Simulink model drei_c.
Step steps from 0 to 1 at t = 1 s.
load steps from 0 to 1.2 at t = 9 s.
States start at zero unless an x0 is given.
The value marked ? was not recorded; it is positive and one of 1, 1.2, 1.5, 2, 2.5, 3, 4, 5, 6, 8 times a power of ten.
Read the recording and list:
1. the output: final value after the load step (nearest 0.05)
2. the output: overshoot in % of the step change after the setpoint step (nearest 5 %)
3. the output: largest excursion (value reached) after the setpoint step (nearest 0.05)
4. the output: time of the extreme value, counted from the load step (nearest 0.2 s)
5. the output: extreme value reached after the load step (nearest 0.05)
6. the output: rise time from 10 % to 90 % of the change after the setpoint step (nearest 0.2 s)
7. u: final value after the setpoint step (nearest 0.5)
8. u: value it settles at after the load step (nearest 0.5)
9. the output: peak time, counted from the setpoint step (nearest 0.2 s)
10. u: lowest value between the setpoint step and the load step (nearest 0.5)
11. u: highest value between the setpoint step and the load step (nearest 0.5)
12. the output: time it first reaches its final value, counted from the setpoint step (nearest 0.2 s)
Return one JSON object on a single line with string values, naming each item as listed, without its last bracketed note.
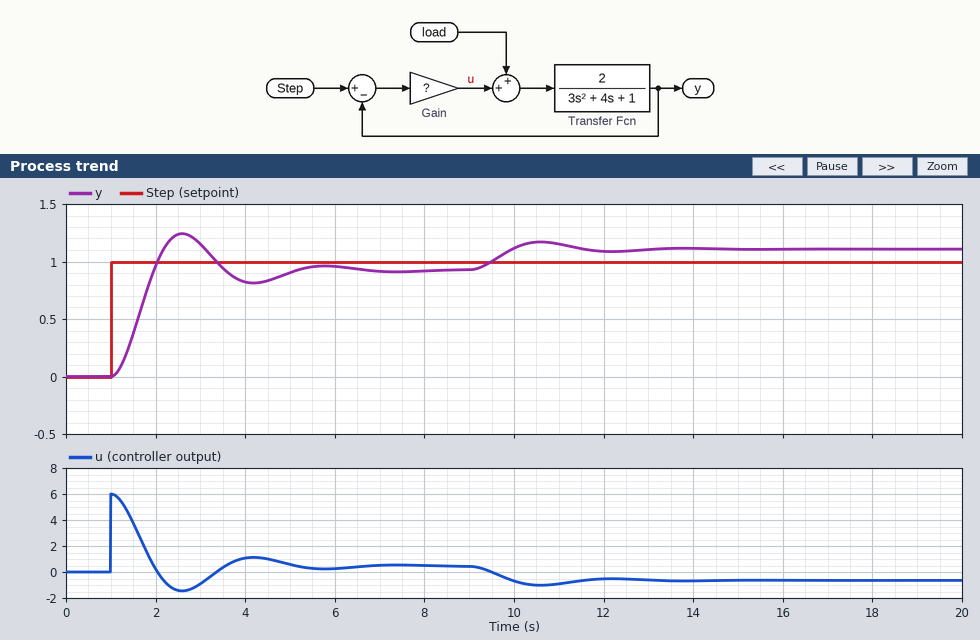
{"the output: final value after the load step": "1.10", "the output: overshoot in % of the step change after the setpoint step": "35 %", "the output: largest excursion (value reached) after the setpoint step": "1.25", "the output: time of the extreme value, counted from the load step": "1.6 s", "the output: extreme value reached after the load step": "1.15", "the output: rise time from 10 % to 90 % of the change after the setpoint step": "0.6 s", "u: final value after the setpoint step": "0.5", "u: value it settles at after the load step": "-0.5", "the output: peak time, counted from the setpoint step": "1.6 s", "u: lowest value between the setpoint step and the load step": "-1.5", "u: highest value between the setpoint step and the load step": "6.0", "the output: time it first reaches its final value, counted from the setpoint step": "1.0 s"}
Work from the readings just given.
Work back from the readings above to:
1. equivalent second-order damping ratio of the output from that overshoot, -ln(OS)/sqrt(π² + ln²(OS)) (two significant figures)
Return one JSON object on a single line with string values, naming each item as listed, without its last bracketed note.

{"equivalent second-order damping ratio of the output from that overshoot, -ln(OS)/sqrt(π² + ln²(OS))": "0.32"}
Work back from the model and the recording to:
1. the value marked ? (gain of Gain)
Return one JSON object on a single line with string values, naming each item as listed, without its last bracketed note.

{"the value marked ?": "6"}
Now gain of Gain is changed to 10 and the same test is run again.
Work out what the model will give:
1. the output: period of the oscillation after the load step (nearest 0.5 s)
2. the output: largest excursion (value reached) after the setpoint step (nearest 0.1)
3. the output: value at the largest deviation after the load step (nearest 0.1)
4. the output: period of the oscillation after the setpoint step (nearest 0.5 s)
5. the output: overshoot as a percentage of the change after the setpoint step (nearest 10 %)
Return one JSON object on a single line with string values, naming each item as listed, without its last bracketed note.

{"the output: period of the oscillation after the load step": "2.5 s", "the output: largest excursion (value reached) after the setpoint step": "1.4", "the output: value at the largest deviation after the load step": "1.1", "the output: period of the oscillation after the setpoint step": "2.5 s", "the output: overshoot as a percentage of the change after the setpoint step": "40 %"}
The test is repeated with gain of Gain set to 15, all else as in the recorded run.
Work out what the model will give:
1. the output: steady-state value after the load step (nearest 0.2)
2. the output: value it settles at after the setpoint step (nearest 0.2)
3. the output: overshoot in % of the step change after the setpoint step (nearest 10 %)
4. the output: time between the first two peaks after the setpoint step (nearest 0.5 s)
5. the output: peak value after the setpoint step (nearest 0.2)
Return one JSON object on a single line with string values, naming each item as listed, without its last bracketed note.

{"the output: steady-state value after the load step": "1.0", "the output: value it settles at after the setpoint step": "1.0", "the output: overshoot in % of the step change after the setpoint step": "50 %", "the output: time between the first two peaks after the setpoint step": "2.0 s", "the output: peak value after the setpoint step": "1.4"}
